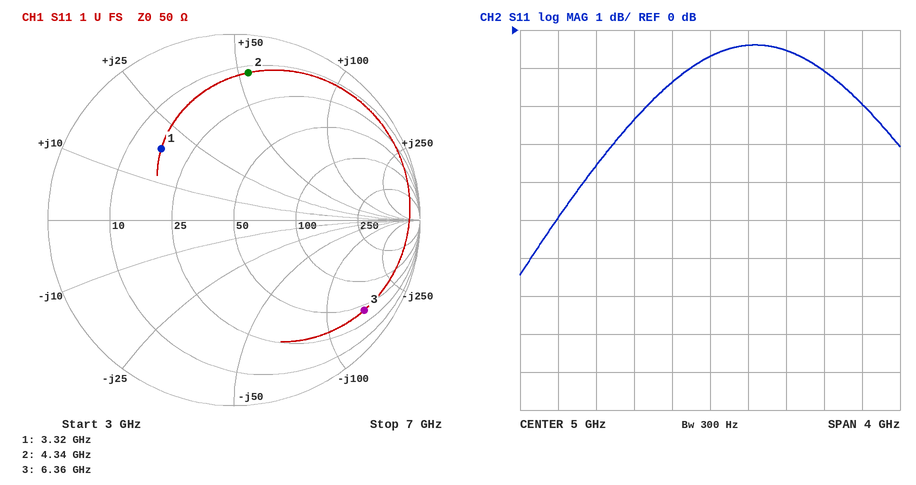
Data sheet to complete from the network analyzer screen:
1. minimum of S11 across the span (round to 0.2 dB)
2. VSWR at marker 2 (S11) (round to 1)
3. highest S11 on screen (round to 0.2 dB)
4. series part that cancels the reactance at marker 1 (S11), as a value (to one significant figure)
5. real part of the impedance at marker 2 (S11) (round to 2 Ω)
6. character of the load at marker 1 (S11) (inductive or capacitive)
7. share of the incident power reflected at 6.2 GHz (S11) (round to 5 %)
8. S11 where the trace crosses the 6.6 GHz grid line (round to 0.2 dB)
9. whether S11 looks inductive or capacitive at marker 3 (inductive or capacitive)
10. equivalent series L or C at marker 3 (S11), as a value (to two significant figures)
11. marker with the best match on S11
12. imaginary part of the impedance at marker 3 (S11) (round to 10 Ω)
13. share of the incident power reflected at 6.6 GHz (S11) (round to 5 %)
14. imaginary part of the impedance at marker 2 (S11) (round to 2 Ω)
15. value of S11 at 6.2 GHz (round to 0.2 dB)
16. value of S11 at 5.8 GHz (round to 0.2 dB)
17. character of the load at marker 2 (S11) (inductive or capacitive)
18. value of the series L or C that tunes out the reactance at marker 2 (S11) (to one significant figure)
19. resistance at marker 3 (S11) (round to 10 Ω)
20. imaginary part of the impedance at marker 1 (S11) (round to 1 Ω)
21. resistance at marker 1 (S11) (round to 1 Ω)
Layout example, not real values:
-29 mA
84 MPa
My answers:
-6.4 dB
9
-0.4 dB
3 pF
12 Ω
inductive
80 %
-2.0 dB
capacitive
170 fF
marker 1
-150 Ω
65 %
+54 Ω
-1.0 dB
-0.6 dB
inductive
700 fF
40 Ω
+18 Ω
17 Ω
